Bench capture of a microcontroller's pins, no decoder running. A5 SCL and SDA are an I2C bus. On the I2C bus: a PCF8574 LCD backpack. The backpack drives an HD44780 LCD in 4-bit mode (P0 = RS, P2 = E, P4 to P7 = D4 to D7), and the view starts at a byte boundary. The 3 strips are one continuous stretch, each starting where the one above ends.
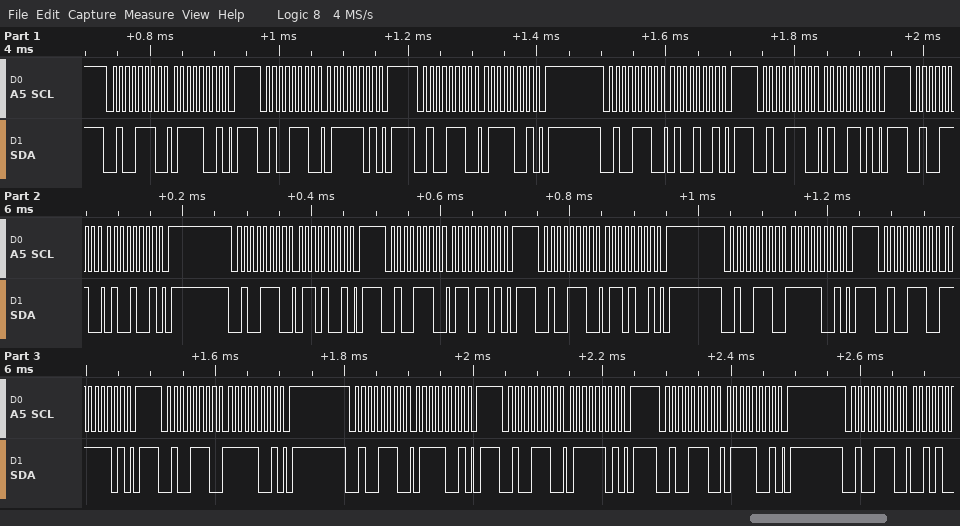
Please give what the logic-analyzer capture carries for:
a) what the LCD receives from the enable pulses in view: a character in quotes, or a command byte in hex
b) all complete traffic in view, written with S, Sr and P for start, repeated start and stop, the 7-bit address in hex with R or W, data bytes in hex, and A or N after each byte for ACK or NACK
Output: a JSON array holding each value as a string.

["'t' 'o'", "S 27W A 79 A P S 27W A 7D A P S 27W A 79 A P S 27W A 49 A P S 27W A 4D A P S 27W A 49 A P S 27W A 69 A P S 27W A 6D A P S 27W A 69 A P S 27W A F9 A P S 27W A FD A P S 27W A F9 A P S 27W A 79 A P S 27W A 7D A P S 27W A 79 A P S 27W A"]
